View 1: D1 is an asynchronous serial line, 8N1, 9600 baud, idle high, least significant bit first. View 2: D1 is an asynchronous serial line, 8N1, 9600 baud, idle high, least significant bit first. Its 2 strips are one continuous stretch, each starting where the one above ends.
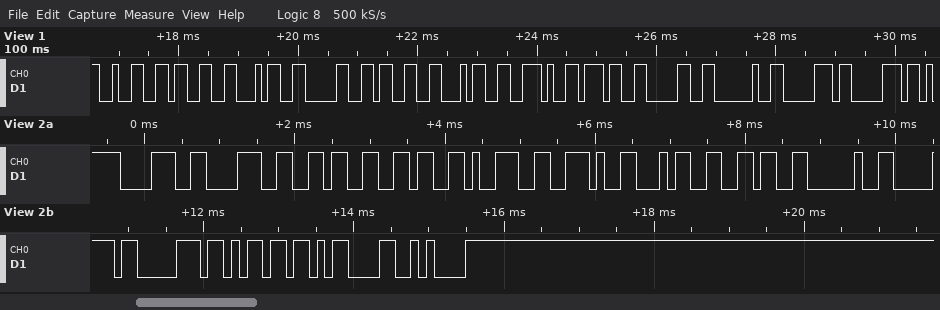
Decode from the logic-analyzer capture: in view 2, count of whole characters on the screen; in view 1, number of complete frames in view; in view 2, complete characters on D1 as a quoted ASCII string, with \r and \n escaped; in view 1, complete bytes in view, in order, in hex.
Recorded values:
14
12
"88669.46 ppm\r\n"
32 33 34 30 33 34 2E 37 30 20 70 70
